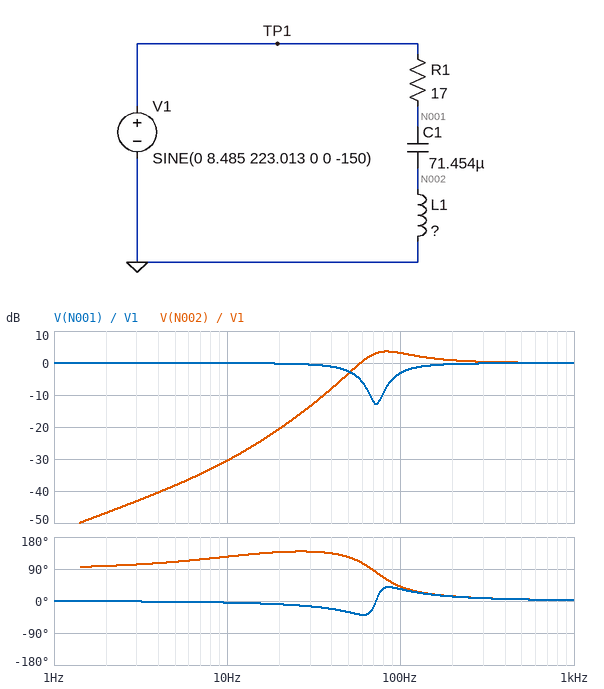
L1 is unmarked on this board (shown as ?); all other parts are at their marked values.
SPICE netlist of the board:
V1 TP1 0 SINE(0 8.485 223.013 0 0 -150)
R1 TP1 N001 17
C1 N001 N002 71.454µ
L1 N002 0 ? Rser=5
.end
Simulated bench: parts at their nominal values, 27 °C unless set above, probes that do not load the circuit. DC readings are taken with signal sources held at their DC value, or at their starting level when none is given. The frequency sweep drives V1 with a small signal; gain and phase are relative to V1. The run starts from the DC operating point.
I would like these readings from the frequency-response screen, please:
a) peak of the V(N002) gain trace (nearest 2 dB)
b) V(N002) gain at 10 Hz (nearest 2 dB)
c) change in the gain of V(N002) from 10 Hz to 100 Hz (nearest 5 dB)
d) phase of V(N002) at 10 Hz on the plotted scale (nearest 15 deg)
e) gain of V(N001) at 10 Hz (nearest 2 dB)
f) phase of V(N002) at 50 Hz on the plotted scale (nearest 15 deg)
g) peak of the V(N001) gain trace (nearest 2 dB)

4 dB
-30 dB
35 dB
120 deg
0 dB
120 deg
0 dB
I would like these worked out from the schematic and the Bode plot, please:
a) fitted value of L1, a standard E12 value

68 mH
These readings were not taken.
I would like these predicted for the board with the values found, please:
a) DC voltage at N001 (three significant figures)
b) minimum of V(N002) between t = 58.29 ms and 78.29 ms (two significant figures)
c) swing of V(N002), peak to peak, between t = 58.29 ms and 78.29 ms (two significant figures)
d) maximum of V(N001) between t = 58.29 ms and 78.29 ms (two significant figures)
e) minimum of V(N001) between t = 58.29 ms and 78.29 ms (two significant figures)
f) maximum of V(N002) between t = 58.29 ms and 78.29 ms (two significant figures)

-4.24 V
-9.2 V
18 V
8.2 V
-8.2 V
9.2 V
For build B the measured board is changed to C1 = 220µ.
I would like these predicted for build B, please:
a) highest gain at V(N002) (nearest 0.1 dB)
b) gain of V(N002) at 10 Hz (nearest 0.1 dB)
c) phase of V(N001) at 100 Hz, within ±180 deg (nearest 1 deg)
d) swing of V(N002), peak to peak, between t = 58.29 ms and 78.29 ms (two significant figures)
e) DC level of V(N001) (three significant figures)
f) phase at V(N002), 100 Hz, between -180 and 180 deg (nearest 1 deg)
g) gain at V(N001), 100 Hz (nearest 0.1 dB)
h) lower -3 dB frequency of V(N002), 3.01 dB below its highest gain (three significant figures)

0.3 dB
-20.7 dB
24 deg
17 V
-4.24 V
25 deg
-1.3 dB
36.5 Hz
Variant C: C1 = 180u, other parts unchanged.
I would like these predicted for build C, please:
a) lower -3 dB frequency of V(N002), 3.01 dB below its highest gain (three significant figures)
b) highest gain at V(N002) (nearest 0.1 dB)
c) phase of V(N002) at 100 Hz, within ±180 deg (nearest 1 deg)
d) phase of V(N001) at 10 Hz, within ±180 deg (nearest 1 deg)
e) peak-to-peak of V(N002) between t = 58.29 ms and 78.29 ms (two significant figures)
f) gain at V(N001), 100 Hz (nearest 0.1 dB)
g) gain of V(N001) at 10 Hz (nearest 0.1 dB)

39.2 Hz
0.7 dB
26 deg
-11 deg
17 V
-1.4 dB
-0.3 dB
